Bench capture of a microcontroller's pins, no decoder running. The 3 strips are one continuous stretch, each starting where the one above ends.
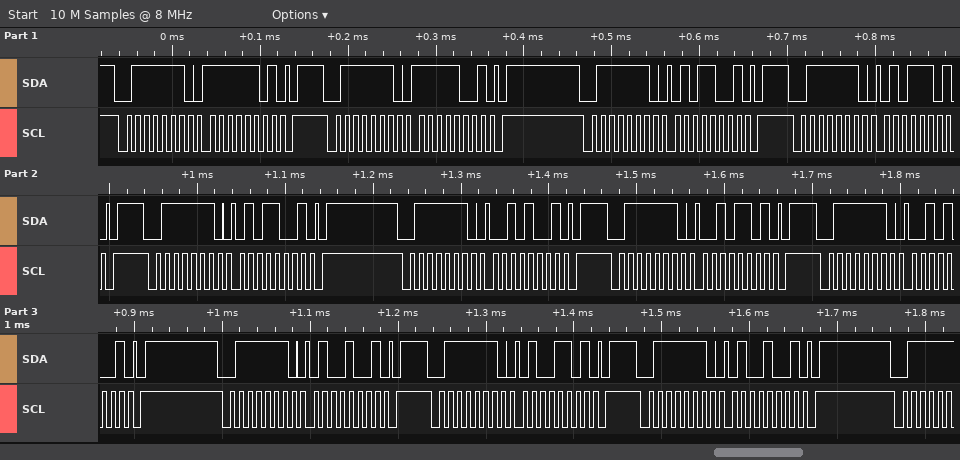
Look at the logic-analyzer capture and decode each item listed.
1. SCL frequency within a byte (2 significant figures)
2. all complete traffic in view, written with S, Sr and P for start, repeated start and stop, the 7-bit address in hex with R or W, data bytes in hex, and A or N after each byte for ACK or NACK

100 kHz
S 3FW A FD A P S 3FW A F9 A P S 3FW A 59 A P S 3FW A 5D A P S 3FW A 59 A P S 3FW A 29 A P S 3FW A 2D A P S 3FW A 29 A P S 3FW A 49 A P S 3FW A 4D A P S 3FW A 49 A P
